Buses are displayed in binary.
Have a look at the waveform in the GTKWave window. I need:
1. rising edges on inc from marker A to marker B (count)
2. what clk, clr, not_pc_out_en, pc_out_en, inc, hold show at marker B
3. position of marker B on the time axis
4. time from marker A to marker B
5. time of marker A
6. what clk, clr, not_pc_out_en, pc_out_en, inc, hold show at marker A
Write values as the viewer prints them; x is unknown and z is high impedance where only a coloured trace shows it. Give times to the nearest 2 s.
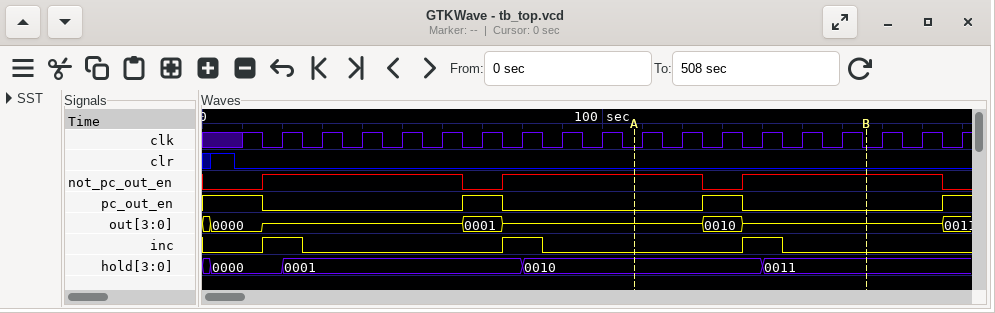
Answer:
1
clk=0, clr=0, not_pc_out_en=1, pc_out_en=0, inc=0, hold=0011
166 s
58 s
108 s
clk=0, clr=0, not_pc_out_en=1, pc_out_en=0, inc=0, hold=0010
